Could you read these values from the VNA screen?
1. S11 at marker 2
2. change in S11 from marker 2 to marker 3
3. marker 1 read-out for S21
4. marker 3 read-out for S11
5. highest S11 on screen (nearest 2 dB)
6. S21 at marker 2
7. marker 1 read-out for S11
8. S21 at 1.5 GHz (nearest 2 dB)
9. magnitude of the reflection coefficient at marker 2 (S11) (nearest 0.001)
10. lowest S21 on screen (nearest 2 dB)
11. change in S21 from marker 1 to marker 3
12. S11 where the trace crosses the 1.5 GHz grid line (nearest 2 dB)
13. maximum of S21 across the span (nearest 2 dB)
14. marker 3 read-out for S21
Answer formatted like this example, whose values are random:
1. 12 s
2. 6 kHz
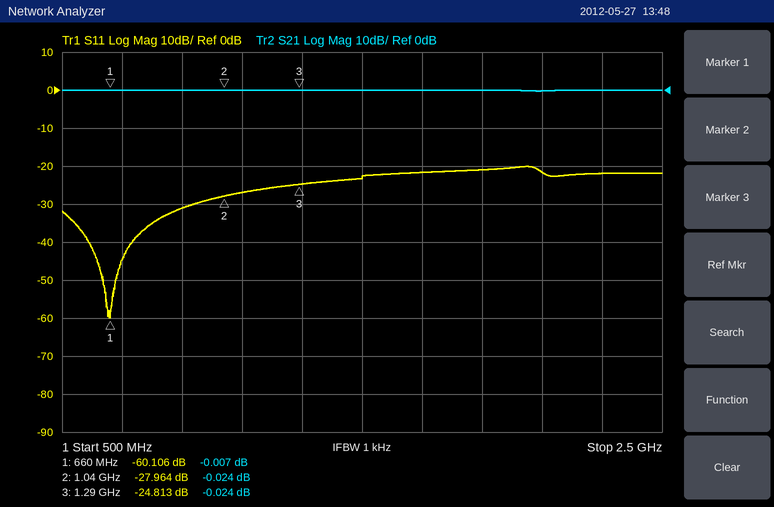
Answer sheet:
1. -27.964 dB
2. 3.151 dB
3. -0.007 dB
4. -24.813 dB
5. -20 dB
6. -0.024 dB
7. -60.106 dB
8. 0 dB
9. 0.040
10. 0 dB
11. -0.017 dB
12. -24 dB
13. 0 dB
14. -0.024 dB
